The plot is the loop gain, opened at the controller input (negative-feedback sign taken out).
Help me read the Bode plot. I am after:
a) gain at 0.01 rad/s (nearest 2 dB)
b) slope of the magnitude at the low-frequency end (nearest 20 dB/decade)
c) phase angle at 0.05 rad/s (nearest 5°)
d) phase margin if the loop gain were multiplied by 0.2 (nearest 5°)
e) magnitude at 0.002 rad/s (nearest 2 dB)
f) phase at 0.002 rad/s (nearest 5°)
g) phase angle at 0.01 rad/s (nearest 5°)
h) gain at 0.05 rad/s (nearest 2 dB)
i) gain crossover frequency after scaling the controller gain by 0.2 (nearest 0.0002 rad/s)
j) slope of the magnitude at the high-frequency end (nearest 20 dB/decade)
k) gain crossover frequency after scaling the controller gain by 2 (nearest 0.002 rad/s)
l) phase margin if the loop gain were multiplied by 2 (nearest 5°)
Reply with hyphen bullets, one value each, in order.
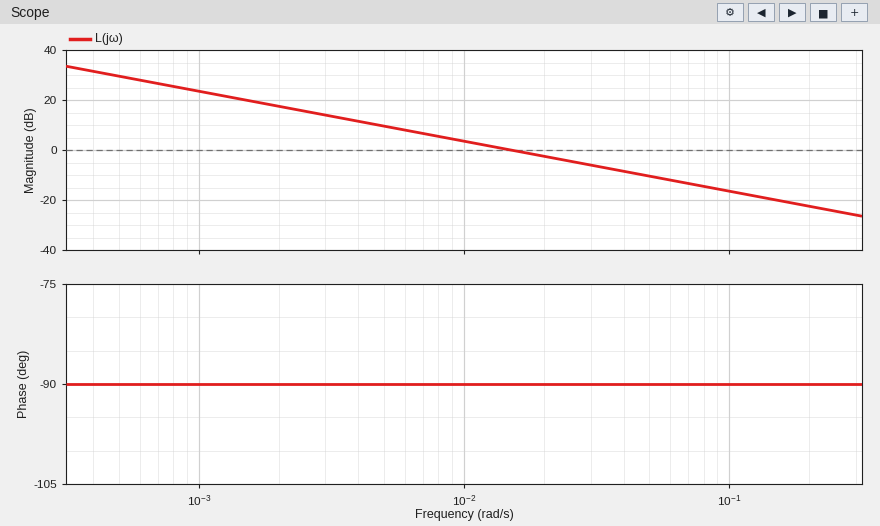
- 4 dB
- -20 dB/decade
- -90°
- 90°
- 18 dB
- -90°
- -90°
- -10 dB
- 0.0030 rad/s
- -20 dB/decade
- 0.030 rad/s
- 90°
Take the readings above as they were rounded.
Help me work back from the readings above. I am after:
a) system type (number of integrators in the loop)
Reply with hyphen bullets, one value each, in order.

- 1
